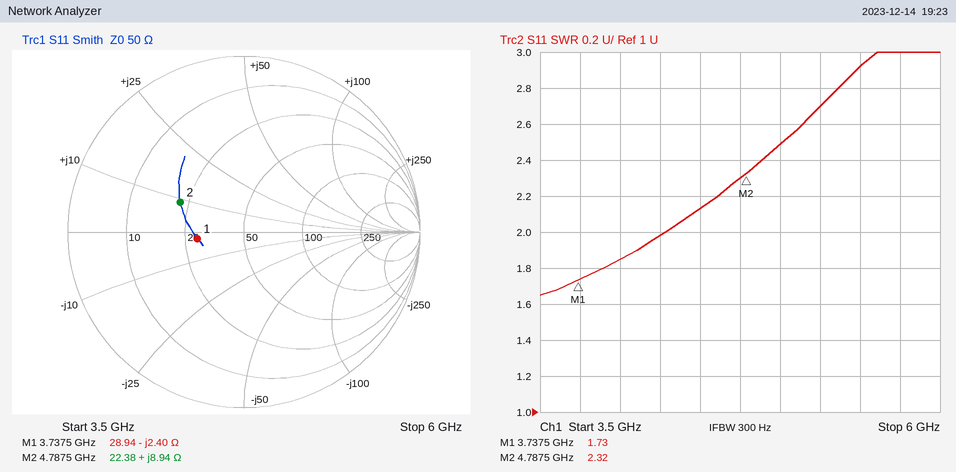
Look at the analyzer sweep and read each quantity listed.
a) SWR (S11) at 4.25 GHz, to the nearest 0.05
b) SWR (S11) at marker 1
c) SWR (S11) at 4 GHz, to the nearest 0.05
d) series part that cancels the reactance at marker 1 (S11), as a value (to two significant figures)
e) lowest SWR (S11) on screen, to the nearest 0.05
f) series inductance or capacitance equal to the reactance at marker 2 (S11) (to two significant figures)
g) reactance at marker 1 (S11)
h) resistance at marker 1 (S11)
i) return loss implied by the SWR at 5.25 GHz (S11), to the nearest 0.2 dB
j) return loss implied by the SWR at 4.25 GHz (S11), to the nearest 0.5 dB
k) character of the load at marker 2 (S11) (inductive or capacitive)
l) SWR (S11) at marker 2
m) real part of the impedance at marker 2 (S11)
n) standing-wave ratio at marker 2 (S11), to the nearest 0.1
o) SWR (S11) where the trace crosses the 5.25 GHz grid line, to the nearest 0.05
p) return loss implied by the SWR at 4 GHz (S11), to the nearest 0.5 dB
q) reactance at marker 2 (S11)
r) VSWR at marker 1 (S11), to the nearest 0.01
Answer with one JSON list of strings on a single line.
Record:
["2.00", "1.73", "1.85", "100 pH", "1.65", "300 pH", "-2.40 Ω", "28.94 Ω", "6.8 dB", "9.5 dB", "inductive", "2.32", "22.38 Ω", "2.3", "2.70", "10.5 dB", "+8.94 Ω", "1.73"]
